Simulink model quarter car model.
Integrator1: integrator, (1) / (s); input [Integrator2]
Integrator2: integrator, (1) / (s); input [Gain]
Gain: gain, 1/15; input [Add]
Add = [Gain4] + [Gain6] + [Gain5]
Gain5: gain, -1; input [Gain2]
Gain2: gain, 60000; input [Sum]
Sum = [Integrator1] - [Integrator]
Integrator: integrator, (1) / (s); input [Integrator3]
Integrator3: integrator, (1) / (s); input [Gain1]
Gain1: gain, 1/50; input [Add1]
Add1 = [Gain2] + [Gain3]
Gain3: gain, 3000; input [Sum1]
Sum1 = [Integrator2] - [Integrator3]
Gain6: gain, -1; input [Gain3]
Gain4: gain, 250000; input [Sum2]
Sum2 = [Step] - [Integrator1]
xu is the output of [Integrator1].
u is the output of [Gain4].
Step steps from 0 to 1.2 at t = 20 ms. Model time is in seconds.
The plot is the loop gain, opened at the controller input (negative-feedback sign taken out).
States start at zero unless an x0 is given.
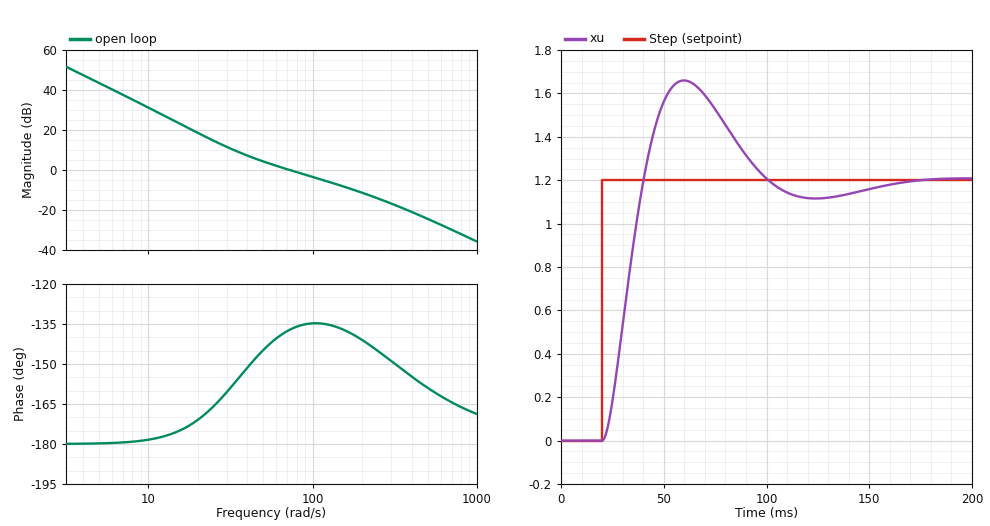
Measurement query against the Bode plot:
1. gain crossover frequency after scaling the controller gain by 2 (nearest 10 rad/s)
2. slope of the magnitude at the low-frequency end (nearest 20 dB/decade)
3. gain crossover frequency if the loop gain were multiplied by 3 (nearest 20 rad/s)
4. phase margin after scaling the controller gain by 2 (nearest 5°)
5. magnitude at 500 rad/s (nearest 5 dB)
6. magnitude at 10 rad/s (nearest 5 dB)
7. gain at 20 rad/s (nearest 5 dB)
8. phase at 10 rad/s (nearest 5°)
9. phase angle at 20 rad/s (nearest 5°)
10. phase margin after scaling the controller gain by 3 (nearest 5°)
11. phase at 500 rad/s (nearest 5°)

130 rad/s
-40 dB/decade
180 rad/s
45°
-25 dB
30 dB
20 dB
-180°
-170°
40°
-160°
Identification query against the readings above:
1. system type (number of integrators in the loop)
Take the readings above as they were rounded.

2
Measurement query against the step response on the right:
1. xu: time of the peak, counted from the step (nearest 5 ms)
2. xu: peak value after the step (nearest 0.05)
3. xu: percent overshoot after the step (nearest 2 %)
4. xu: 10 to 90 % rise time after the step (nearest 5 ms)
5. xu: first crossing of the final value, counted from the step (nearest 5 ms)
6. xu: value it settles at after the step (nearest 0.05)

40 ms
1.65
38 %
15 ms
20 ms
1.20
